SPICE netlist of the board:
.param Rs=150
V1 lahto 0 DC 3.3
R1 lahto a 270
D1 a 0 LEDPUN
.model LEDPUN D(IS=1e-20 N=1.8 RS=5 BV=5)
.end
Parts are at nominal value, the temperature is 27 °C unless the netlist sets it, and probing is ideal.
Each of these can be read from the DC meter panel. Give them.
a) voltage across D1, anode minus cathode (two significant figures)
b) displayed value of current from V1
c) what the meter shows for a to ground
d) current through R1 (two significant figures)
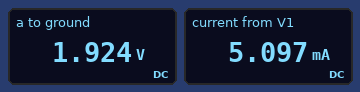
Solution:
1.9 V
5.097 mA
1.924 V
5.1 mA
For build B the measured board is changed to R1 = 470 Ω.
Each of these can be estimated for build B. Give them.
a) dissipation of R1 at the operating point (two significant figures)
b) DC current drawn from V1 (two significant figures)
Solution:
4.2 mW
3.0 mA
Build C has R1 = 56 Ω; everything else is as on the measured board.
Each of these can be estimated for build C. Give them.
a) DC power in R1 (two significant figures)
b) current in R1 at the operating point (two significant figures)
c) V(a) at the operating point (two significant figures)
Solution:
27 mW
22 mA
2.1 V
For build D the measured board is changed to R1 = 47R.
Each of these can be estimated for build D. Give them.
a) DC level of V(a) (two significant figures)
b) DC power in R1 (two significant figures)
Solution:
2.1 V
31 mW
